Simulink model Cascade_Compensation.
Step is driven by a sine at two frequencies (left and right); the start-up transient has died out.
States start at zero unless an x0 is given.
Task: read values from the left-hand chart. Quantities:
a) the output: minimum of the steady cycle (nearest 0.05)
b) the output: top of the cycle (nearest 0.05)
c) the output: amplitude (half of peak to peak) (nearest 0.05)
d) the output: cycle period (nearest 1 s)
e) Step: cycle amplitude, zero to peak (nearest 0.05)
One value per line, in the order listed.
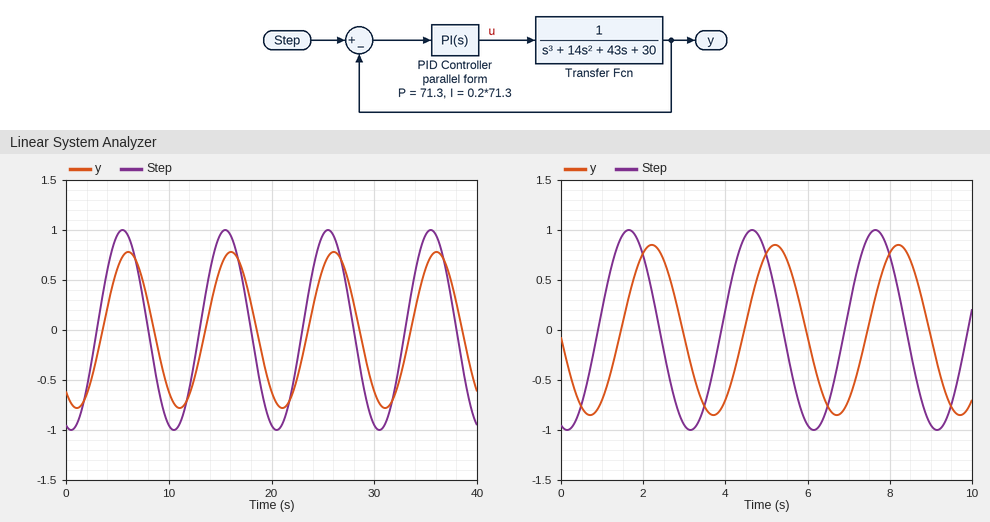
-0.80
0.80
0.80
10 s
1.00
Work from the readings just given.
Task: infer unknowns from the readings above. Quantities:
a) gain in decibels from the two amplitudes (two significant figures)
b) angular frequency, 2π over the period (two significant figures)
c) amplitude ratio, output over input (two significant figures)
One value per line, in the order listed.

-1.9 dB
0.63 rad/s
0.80
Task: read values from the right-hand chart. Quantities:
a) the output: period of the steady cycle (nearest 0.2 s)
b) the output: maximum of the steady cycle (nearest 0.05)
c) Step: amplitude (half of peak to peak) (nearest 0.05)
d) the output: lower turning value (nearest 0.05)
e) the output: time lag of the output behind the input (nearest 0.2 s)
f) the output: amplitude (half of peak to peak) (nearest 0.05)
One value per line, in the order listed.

3.0 s
0.85
1.00
-0.85
0.6 s
0.85
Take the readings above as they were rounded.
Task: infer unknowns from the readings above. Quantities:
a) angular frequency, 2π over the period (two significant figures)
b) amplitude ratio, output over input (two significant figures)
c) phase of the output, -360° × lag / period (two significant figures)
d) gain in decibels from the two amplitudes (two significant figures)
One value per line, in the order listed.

2.1 rad/s
0.85
-72°
-1.4 dB
